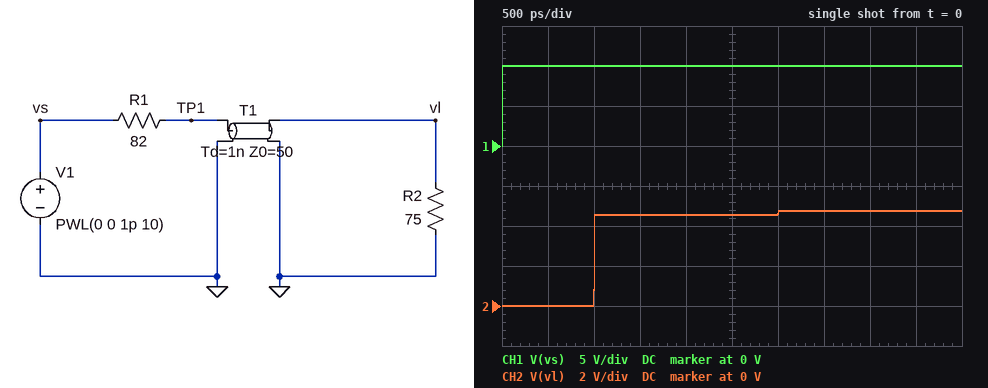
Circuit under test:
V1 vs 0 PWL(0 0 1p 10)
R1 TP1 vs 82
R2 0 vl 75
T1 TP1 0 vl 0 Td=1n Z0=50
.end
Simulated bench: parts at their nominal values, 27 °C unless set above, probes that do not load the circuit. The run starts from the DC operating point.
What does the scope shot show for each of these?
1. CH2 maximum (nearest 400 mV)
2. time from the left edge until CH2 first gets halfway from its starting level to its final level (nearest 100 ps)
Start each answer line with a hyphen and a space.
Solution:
- 4.8 V
- 1.0 ns
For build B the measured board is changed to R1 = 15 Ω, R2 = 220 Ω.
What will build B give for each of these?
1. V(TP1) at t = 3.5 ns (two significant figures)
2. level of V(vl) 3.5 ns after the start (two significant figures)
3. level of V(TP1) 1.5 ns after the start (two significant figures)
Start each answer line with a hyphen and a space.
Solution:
- 9.9 V
- 8.3 V
- 7.7 V
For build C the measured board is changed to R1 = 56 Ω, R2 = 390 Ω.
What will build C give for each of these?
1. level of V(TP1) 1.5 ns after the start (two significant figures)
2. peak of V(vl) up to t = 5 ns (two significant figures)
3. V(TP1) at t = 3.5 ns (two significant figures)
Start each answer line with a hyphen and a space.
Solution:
- 4.7 V
- 8.7 V
- 8.6 V
